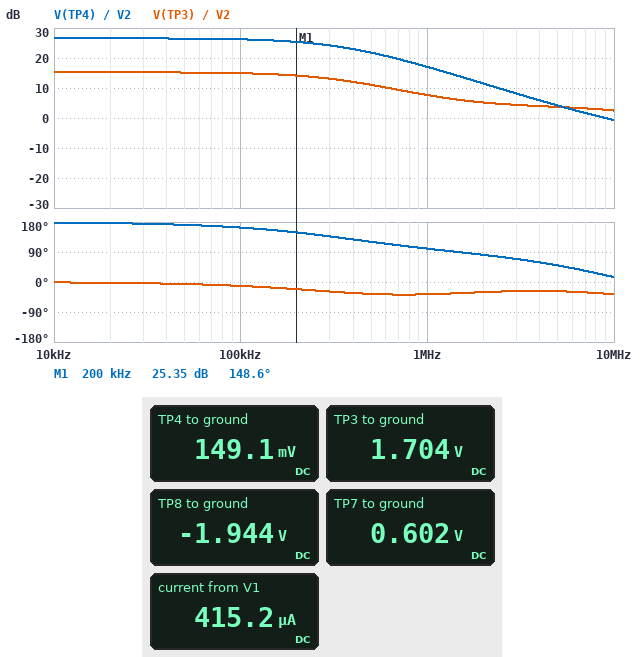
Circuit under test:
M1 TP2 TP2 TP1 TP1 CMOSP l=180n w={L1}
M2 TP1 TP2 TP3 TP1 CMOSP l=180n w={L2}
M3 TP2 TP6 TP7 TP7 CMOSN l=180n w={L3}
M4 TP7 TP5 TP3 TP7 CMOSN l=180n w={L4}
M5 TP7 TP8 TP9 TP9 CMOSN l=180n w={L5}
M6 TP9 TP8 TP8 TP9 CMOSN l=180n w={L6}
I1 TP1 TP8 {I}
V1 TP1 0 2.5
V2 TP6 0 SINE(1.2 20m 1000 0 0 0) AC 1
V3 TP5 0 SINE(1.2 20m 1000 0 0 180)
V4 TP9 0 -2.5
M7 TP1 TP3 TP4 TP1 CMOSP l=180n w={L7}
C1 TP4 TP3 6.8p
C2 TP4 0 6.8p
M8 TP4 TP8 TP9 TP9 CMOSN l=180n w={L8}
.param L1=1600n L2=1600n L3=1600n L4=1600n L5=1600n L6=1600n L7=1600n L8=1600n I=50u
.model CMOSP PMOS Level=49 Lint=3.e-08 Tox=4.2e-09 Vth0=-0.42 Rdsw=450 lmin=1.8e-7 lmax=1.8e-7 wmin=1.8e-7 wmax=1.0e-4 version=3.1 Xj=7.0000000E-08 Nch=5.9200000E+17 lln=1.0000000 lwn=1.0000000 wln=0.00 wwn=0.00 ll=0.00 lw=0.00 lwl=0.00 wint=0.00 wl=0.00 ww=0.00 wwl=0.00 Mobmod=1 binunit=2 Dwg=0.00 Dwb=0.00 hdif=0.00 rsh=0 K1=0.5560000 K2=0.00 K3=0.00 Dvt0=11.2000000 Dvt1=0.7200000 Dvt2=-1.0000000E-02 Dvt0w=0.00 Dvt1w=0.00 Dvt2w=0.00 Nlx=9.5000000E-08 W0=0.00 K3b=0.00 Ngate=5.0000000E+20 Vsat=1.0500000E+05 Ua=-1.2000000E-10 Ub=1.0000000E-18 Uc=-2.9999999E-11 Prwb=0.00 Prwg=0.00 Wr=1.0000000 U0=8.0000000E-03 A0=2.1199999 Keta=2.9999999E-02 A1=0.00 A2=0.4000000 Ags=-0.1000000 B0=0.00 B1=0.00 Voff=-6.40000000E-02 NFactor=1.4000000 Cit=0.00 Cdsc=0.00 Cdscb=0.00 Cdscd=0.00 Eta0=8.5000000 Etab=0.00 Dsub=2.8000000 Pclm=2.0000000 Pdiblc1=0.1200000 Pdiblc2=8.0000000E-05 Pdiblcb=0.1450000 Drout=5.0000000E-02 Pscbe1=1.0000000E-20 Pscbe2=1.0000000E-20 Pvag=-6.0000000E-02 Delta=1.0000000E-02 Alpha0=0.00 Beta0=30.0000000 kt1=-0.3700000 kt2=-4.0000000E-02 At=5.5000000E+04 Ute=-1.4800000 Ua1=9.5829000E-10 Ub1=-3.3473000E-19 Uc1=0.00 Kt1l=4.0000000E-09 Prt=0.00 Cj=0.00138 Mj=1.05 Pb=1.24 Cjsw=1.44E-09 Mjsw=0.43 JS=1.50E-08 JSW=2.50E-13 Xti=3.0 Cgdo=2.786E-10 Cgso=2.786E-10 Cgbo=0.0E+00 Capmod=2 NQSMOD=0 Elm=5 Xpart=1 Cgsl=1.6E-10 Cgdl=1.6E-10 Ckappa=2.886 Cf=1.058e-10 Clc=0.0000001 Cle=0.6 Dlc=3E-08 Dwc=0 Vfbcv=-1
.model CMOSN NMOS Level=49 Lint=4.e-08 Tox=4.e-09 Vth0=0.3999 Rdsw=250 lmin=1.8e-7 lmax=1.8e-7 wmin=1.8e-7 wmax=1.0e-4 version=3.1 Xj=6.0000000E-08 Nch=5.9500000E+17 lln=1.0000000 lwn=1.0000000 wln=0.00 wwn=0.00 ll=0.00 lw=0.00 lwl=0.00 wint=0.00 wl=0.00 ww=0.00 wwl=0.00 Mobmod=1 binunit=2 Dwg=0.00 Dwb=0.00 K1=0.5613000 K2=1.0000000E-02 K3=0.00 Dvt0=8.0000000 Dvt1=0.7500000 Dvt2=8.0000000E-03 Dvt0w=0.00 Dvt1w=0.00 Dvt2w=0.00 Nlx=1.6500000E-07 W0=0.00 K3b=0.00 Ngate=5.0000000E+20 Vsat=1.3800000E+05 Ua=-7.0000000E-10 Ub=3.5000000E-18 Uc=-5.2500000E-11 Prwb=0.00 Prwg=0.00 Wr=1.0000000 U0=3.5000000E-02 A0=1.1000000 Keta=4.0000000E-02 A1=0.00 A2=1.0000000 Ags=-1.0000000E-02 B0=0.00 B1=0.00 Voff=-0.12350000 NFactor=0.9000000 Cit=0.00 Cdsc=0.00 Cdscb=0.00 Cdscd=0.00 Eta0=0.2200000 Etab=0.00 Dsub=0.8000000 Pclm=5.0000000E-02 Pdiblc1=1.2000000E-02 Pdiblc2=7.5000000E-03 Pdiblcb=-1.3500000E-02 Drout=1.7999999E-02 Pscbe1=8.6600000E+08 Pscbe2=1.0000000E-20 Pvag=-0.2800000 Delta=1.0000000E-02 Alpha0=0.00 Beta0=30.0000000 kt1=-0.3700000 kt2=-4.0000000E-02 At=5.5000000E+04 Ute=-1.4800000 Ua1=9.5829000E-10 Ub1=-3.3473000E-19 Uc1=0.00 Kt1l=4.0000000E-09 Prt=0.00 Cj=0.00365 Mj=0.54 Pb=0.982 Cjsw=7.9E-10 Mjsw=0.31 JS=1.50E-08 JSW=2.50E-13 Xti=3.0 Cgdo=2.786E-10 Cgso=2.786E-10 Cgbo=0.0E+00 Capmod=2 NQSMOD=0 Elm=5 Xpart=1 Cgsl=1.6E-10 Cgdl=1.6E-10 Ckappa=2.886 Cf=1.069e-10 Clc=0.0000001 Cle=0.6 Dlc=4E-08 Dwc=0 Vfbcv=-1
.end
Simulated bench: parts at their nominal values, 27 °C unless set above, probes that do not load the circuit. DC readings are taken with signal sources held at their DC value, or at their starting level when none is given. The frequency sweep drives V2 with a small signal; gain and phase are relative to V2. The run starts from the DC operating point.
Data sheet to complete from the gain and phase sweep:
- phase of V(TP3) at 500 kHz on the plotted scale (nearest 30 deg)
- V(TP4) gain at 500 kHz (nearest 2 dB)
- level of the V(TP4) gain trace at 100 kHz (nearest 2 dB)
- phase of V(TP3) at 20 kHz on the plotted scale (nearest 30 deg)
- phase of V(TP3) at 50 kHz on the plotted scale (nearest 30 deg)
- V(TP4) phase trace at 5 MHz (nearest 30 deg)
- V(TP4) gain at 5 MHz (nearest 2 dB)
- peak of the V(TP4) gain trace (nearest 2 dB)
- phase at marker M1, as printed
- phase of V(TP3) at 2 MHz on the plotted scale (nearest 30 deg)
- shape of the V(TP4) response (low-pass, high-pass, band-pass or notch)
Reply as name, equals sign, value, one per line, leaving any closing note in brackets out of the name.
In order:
phase of V(TP3) at 500 kHz on the plotted scale = -30 deg
V(TP4) gain at 500 kHz = 22 dB
level of the V(TP4) gain trace at 100 kHz = 26 dB
phase of V(TP3) at 20 kHz on the plotted scale = 0 deg
phase of V(TP3) at 50 kHz on the plotted scale = 0 deg
V(TP4) phase trace at 5 MHz = 60 deg
V(TP4) gain at 5 MHz = 4 dB
peak of the V(TP4) gain trace = 26 dB
phase at marker M1, as printed = 148.6 deg
phase of V(TP3) at 2 MHz on the plotted scale = -30 deg
shape of the V(TP4) response = low-pass
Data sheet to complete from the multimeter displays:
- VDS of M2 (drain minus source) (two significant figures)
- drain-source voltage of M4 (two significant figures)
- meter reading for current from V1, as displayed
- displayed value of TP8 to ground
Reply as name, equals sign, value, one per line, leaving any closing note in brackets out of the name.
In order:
VDS of M2 (drain minus source) = 800 mV
drain-source voltage of M4 = -1.1 V
meter reading for current from V1, as displayed = 415.2 µA
displayed value of TP8 to ground = -1.944 V
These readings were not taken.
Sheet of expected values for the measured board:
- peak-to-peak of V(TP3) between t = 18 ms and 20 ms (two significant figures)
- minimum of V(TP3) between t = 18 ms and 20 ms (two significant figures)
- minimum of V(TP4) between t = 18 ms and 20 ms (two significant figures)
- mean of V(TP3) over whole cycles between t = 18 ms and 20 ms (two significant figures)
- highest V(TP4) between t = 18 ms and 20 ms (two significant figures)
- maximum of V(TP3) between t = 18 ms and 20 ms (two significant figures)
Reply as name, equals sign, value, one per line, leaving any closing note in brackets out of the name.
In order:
peak-to-peak of V(TP3) between t = 18 ms and 20 ms = 460 mV
minimum of V(TP3) between t = 18 ms and 20 ms = 1.5 V
minimum of V(TP4) between t = 18 ms and 20 ms = -870 mV
mean of V(TP3) over whole cycles between t = 18 ms and 20 ms = 1.7 V
highest V(TP4) between t = 18 ms and 20 ms = 900 mV
maximum of V(TP3) between t = 18 ms and 20 ms = 1.9 V
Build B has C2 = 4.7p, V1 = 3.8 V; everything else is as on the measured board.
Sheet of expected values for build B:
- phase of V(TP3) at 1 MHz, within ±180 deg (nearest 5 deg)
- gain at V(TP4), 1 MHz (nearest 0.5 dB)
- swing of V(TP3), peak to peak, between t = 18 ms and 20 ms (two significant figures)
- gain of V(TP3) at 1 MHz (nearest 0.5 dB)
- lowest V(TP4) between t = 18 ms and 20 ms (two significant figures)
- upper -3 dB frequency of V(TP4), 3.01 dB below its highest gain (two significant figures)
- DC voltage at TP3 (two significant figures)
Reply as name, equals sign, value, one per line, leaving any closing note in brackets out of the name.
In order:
phase of V(TP3) at 1 MHz, within ±180 deg = -40 deg
gain at V(TP4), 1 MHz = 18.5 dB
swing of V(TP3), peak to peak, between t = 18 ms and 20 ms = 500 mV
gain of V(TP3) at 1 MHz = 8.0 dB
lowest V(TP4) between t = 18 ms and 20 ms = -530 mV
upper -3 dB frequency of V(TP4), 3.01 dB below its highest gain = 360 kHz
DC voltage at TP3 = 3.0 V
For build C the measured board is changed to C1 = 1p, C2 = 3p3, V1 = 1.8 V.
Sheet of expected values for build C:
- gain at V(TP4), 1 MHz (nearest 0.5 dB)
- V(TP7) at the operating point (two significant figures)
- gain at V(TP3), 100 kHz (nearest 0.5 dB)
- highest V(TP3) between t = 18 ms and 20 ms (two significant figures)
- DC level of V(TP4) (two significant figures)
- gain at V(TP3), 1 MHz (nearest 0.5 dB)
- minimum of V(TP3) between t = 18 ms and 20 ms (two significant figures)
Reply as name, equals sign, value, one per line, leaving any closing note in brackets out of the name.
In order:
gain at V(TP4), 1 MHz = 24.5 dB
V(TP7) at the operating point = 550 mV
gain at V(TP3), 100 kHz = 14.5 dB
highest V(TP3) between t = 18 ms and 20 ms = 1.2 V
DC level of V(TP4) = -140 mV
gain at V(TP3), 1 MHz = 14.0 dB
minimum of V(TP3) between t = 18 ms and 20 ms = 800 mV
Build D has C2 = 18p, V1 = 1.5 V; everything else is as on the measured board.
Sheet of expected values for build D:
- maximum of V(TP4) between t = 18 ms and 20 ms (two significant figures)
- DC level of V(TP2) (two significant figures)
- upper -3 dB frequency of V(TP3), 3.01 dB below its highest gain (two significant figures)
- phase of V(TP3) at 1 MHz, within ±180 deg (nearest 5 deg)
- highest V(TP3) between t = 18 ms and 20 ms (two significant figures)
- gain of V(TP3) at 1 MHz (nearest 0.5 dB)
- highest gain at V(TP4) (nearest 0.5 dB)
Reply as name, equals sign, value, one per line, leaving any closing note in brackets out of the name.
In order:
maximum of V(TP4) between t = 18 ms and 20 ms = -67 mV
DC level of V(TP2) = 710 mV
upper -3 dB frequency of V(TP3), 3.01 dB below its highest gain = 730 kHz
phase of V(TP3) at 1 MHz, within ±180 deg = -20 deg
highest V(TP3) between t = 18 ms and 20 ms = 840 mV
gain of V(TP3) at 1 MHz = 3.0 dB
highest gain at V(TP4) = 17.5 dB
